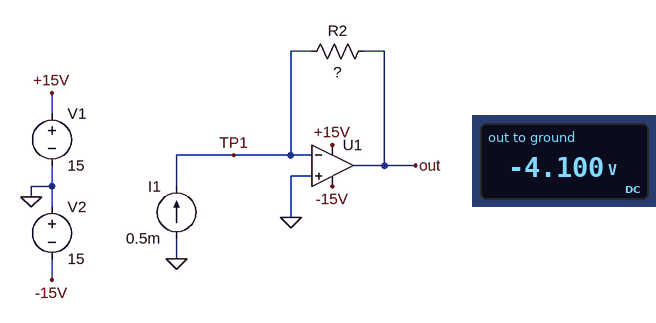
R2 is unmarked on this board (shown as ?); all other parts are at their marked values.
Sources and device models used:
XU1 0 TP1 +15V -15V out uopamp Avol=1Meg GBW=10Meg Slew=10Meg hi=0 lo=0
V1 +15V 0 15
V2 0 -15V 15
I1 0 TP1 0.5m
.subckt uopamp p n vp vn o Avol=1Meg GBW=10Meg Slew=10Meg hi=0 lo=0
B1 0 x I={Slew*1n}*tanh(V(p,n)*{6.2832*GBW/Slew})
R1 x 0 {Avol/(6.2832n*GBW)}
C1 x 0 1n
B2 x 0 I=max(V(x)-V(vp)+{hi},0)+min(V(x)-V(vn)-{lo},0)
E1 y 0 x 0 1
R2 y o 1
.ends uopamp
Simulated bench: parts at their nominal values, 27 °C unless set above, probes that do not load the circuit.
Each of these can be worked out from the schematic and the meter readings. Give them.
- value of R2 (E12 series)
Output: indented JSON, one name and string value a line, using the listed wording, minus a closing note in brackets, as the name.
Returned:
{
  "value of R2": "8.2 kΩ"
}
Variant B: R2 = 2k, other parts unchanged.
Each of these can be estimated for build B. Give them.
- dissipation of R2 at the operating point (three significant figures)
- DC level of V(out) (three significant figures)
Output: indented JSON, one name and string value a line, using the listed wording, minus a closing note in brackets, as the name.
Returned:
{
  "dissipation of R2 at the operating point": "500 µW",
  "DC level of V(out)": "-1.00 V"
}
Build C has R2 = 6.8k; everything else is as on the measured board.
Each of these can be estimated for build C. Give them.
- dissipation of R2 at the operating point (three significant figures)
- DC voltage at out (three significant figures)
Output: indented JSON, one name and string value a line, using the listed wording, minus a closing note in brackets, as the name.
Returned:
{
  "dissipation of R2 at the operating point": "1.70 mW",
  "DC voltage at out": "-3.40 V"
}
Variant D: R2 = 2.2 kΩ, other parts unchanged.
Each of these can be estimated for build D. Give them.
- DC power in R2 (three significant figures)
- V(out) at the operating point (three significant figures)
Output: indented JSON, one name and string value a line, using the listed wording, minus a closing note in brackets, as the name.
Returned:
{
  "DC power in R2": "550 µW",
  "V(out) at the operating point": "-1.10 V"
}
